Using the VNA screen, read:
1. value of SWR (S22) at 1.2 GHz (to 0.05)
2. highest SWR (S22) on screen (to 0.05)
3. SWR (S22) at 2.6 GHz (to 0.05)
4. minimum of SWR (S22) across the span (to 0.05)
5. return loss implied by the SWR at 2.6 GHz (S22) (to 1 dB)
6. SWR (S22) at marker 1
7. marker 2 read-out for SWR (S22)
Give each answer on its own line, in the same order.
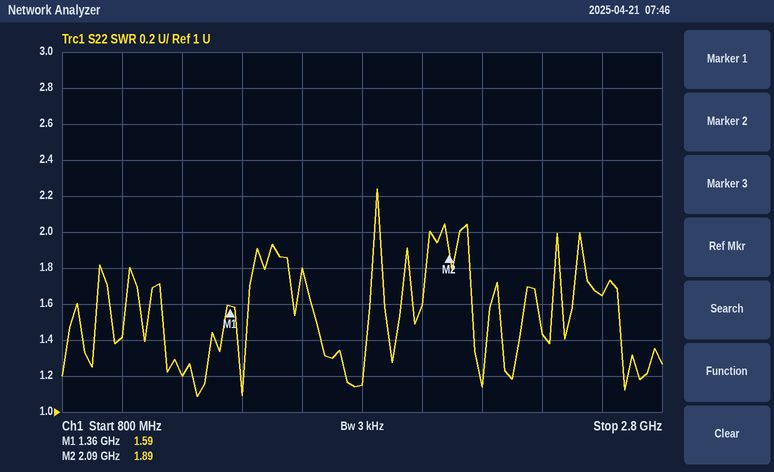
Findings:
1.20
2.25
1.65
1.10
12 dB
1.59
1.89
